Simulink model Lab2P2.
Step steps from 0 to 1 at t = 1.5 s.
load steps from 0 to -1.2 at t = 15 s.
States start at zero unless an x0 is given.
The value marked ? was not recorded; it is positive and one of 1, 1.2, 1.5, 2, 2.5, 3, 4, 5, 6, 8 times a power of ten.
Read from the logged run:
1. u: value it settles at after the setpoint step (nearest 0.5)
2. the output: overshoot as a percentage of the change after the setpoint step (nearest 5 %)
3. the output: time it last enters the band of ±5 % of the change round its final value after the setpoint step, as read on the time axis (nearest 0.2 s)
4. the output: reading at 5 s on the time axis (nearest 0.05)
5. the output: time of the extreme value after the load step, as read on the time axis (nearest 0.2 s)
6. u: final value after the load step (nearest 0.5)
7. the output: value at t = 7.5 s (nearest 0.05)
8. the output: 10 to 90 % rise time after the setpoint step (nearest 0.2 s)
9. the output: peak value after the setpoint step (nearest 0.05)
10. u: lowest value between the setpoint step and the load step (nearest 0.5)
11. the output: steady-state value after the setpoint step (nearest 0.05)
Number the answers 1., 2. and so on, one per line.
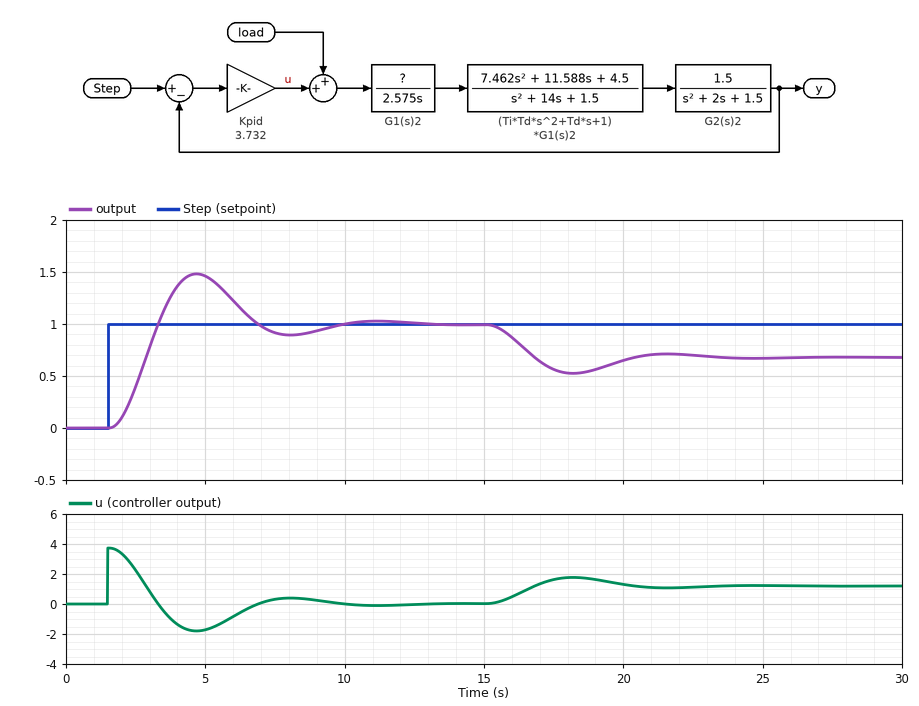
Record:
1. 0.0
2. 50 %
3. 9.2 s
4. 1.45
5. 18.2 s
6. 1.0
7. 0.90
8. 1.2 s
9. 1.50
10. -2.0
11. 1.00
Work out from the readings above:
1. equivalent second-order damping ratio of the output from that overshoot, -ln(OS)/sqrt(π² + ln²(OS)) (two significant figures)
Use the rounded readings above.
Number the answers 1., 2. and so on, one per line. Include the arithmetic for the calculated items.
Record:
1. ln(0.5) = -0.693; 0.693 / sqrt(9.870 + 0.480) = 0.22
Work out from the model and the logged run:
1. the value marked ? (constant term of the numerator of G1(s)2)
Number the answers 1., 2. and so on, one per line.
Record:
1. 1
